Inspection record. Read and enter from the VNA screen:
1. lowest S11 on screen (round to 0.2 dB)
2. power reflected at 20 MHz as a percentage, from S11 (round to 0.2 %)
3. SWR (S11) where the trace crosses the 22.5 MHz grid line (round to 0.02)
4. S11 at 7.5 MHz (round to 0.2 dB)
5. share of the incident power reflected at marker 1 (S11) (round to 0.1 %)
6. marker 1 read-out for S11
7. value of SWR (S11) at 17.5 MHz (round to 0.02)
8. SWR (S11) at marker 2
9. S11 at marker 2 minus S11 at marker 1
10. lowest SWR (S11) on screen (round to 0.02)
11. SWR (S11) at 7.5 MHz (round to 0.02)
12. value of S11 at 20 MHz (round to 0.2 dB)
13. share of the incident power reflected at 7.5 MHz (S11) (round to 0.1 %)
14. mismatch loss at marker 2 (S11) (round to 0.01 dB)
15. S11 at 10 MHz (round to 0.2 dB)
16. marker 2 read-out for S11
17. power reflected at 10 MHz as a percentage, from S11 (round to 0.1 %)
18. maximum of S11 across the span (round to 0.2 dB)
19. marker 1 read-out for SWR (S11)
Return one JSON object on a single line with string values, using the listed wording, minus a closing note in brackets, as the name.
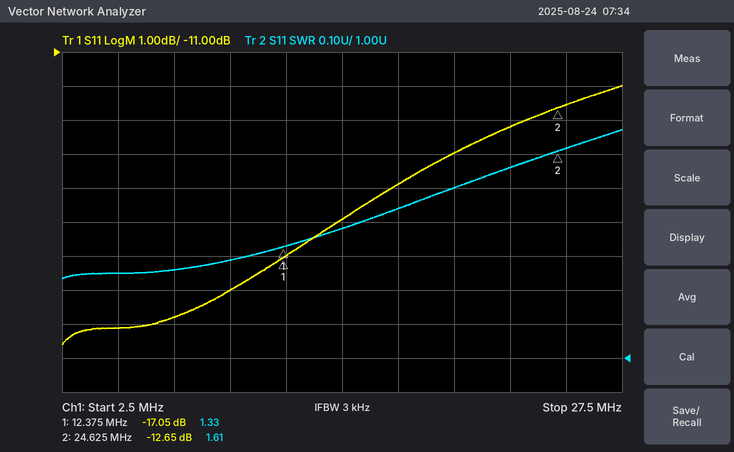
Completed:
{"lowest S11 on screen": "-19.6 dB", "power reflected at 20 MHz as a percentage, from S11": "4.0 %", "SWR (S11) where the trace crosses the 22.5 MHz grid line": "1.56", "S11 at 7.5 MHz": "-18.8 dB", "share of the incident power reflected at marker 1 (S11)": "2.0 %", "marker 1 read-out for S11": "-17.05 dB", "value of SWR (S11) at 17.5 MHz": "1.44", "SWR (S11) at marker 2": "1.61", "S11 at marker 2 minus S11 at marker 1": "4.40 dB", "lowest SWR (S11) on screen": "1.24", "SWR (S11) at 7.5 MHz": "1.26", "value of S11 at 20 MHz": "-14.0 dB", "share of the incident power reflected at 7.5 MHz (S11)": "1.3 %", "mismatch loss at marker 2 (S11)": "0.24 dB", "S11 at 10 MHz": "-18.0 dB", "marker 2 read-out for S11": "-12.65 dB", "power reflected at 10 MHz as a percentage, from S11": "1.6 %", "maximum of S11 across the span": "-12.0 dB", "marker 1 read-out for SWR": "1.33"}
